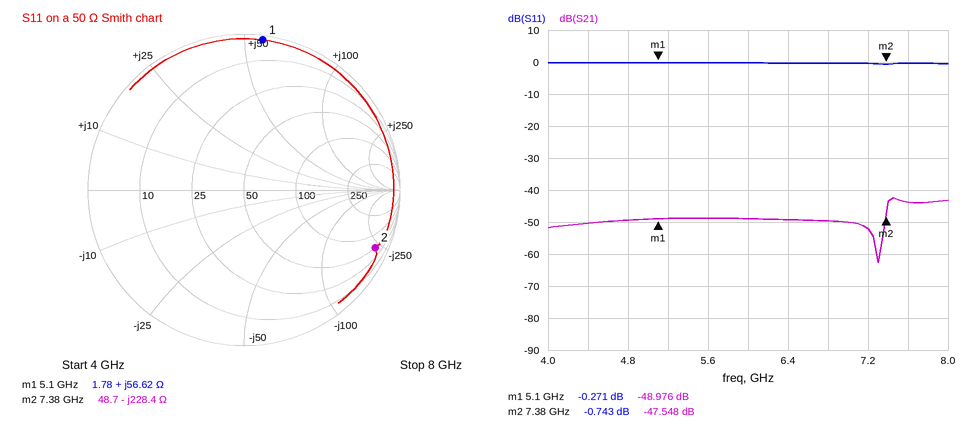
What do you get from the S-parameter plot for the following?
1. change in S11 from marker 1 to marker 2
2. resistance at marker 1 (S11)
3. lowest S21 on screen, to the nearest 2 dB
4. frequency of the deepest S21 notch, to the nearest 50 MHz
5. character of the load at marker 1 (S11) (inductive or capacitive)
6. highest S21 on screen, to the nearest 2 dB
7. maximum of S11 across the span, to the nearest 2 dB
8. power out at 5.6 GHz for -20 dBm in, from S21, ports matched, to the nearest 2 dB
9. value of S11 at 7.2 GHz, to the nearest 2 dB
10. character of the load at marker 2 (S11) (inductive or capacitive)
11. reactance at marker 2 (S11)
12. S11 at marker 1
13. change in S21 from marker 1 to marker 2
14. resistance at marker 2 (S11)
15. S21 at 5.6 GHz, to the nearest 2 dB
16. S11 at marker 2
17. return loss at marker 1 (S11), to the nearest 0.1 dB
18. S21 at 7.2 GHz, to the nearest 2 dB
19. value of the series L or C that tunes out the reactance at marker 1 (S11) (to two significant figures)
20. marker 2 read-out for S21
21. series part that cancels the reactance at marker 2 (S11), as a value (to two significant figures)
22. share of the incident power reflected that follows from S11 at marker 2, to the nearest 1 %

-0.472 dB
1.78 Ω
-62 dB
7.30 GHz
inductive
-42 dB
0 dB
-68 dBm
0 dB
capacitive
-228.4 Ω
-0.271 dB
1.428 dB
48.7 Ω
-48 dB
-0.743 dB
0.3 dB
-52 dB
550 fF
-47.548 dB
4.9 nH
84 %
